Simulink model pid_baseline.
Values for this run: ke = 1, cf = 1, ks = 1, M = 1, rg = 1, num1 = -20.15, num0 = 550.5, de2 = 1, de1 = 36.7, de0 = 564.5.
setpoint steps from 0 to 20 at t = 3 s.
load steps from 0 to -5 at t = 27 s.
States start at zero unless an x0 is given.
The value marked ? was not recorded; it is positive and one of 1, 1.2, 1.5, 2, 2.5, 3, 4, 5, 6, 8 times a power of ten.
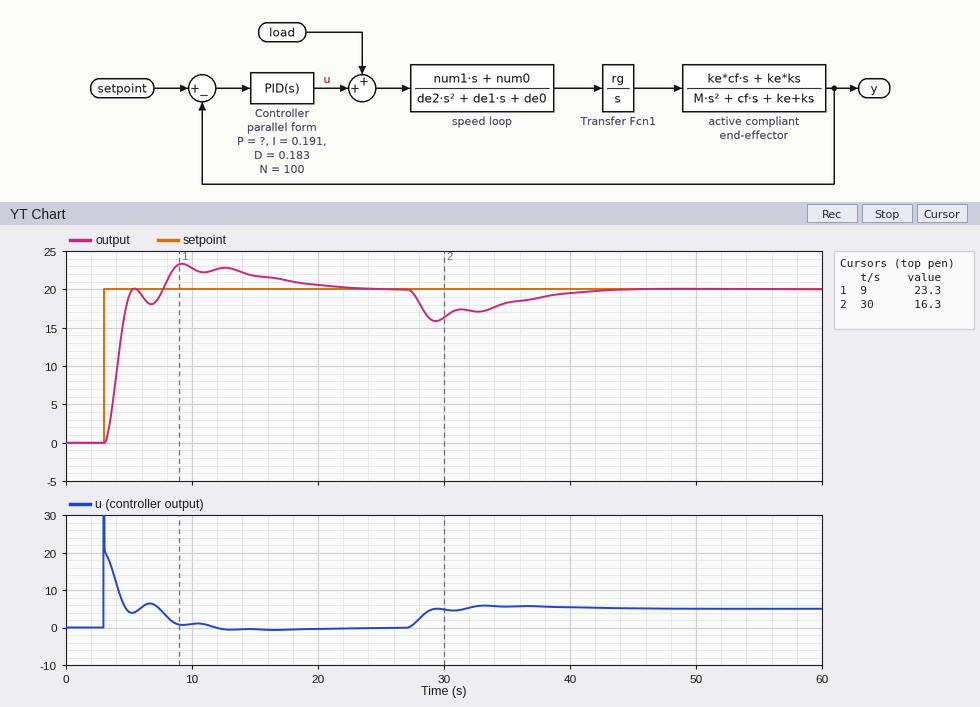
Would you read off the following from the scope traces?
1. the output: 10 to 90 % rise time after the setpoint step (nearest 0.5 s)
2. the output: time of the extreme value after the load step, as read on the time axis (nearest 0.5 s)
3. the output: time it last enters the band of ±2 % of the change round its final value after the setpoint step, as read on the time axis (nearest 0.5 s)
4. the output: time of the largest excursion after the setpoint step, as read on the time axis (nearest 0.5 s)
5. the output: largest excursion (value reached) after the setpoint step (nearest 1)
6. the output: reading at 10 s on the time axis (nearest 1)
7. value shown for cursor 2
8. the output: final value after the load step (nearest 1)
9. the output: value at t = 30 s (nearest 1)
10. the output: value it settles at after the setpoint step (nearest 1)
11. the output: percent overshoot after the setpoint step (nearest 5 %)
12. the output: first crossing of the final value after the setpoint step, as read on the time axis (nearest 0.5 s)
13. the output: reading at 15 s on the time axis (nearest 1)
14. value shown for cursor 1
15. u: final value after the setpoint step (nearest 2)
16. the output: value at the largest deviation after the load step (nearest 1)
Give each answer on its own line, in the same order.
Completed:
1.5 s
29.5 s
21.0 s
9.0 s
23
23
16.3
20
16
20
15 %
5.5 s
22
23.3
0
16
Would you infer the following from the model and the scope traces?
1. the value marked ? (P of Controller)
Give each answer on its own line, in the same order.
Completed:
1
